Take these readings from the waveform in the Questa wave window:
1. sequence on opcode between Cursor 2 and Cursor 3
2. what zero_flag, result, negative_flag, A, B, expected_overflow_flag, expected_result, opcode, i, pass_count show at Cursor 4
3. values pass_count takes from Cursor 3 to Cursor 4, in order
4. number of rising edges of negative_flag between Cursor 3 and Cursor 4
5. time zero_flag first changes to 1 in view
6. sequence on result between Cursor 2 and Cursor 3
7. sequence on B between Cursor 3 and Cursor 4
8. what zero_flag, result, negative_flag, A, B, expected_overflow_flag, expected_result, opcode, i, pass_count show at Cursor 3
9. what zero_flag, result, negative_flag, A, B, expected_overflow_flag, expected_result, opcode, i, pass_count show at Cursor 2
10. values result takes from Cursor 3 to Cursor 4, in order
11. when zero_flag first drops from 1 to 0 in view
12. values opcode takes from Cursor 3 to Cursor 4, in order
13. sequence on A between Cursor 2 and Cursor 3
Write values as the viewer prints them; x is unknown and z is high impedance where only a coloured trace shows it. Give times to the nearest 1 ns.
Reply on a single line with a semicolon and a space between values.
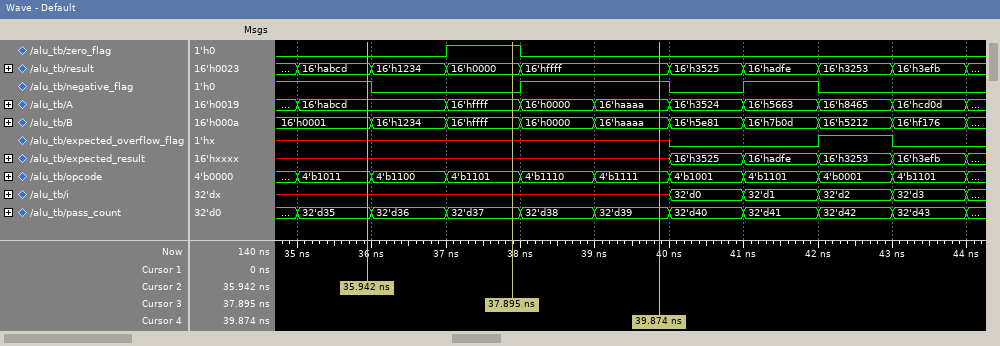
4'b1011, 4'b1100, 4'b1101; zero_flag=0, result=16'hffff, negative_flag=1, A=16'haaaa, B=16'haaaa, expected_overflow_flag=x, expected_result=x, opcode=4'b1111, i=x, pass_count=32'd39; 32'd37, 32'd38, 32'd39; 1; 37 ns; 16'habcd, 16'h1234, 16'h0000; 16'hffff, 16'h0000, 16'haaaa; zero_flag=1, result=16'h0000, negative_flag=0, A=16'hffff, B=16'hffff, expected_overflow_flag=x, expected_result=x, opcode=4'b1101, i=x, pass_count=32'd37; zero_flag=0, result=16'habcd, negative_flag=1, A=16'habcd, B=16'h0001, expected_overflow_flag=x, expected_result=x, opcode=4'b1011, i=x, pass_count=32'd35; 16'h0000, 16'hffff; 38 ns; 4'b1101, 4'b1110, 4'b1111; 16'habcd, 16'hffff
